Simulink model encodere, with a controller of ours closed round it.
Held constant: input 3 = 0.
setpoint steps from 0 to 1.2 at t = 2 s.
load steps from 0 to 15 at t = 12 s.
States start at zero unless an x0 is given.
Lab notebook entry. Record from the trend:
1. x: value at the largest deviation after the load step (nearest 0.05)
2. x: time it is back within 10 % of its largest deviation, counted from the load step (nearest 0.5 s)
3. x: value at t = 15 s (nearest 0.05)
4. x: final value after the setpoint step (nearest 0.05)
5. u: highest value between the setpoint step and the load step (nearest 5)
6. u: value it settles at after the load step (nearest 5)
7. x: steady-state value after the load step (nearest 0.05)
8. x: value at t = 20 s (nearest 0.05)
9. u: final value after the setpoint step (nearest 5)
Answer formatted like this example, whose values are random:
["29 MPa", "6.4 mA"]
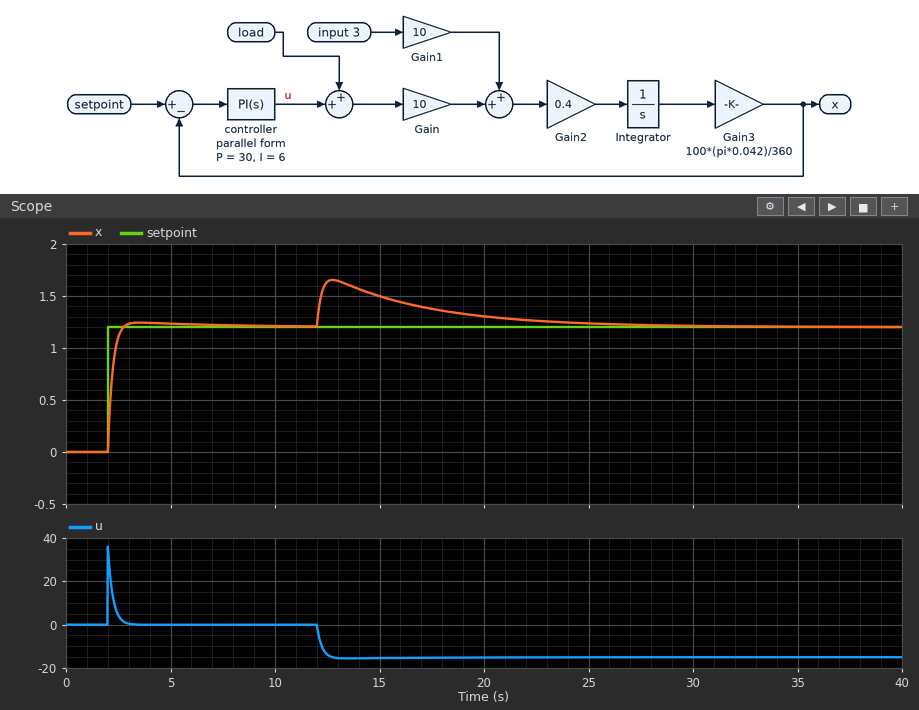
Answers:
["1.65", "12.0 s", "1.50", "1.20", "35", "-15", "1.20", "1.30", "0"]
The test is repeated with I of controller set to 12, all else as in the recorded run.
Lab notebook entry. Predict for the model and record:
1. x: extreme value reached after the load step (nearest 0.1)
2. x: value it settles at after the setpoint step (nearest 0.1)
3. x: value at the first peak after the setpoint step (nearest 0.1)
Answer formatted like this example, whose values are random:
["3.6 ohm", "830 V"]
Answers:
["1.6", "1.2", "1.3"]
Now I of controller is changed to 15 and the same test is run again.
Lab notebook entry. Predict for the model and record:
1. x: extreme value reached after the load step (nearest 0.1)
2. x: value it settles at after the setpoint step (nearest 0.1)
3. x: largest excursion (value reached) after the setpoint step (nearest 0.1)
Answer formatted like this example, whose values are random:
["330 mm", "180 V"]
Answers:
["1.6", "1.2", "1.3"]
